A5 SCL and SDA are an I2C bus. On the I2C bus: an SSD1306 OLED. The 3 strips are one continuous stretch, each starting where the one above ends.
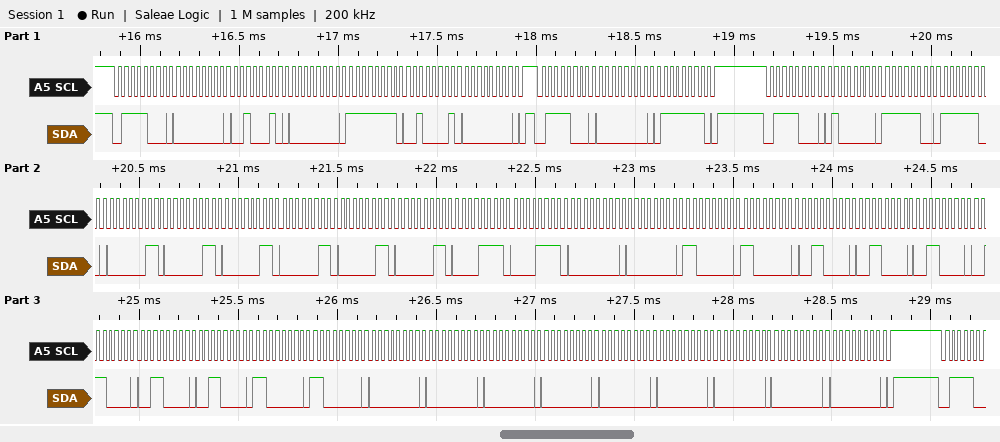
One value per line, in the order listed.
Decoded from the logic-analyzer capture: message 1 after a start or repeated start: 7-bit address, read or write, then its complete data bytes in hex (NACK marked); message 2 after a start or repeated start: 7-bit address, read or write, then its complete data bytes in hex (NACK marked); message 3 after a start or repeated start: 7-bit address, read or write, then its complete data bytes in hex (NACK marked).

0x3C write: 00 22 00 FF 21 00
0x3C write: 00 7F
0x3C write: 40 FC FC 03 03 03 03 03 03 0F 0F 00 00 C0 C0 30 30 30 30 30 30 C0 C0 00 00 00 00 00 00 00 00 00
